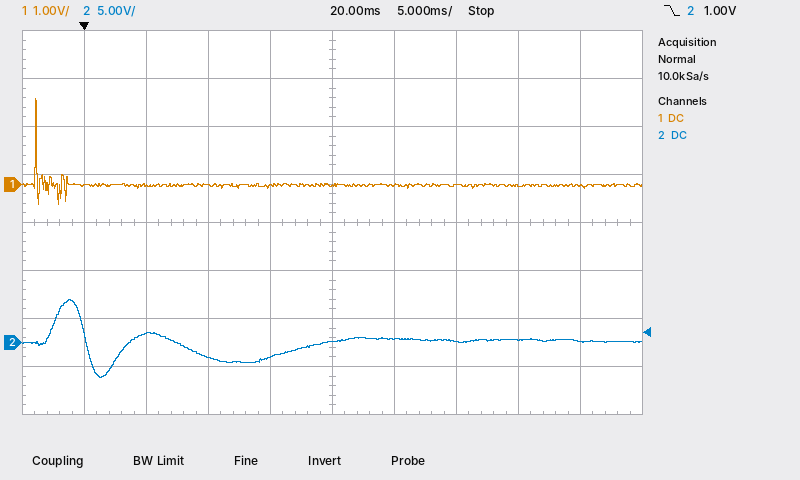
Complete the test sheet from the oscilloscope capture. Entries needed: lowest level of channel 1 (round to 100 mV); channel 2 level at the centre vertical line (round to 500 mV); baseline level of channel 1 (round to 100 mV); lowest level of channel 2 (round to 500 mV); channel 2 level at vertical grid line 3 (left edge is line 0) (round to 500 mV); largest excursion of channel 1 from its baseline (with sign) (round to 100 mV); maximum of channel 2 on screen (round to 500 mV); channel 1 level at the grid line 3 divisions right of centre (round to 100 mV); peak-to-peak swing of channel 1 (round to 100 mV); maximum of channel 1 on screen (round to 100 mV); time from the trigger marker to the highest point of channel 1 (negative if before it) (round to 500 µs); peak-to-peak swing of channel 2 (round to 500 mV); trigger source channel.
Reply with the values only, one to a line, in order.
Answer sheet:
-400 mV
0.0 V
0.0 V
-3.5 V
-1.5 V
+1.8 V
4.5 V
0.0 V
2.2 V
1.8 V
-4.0 ms
8.0 V
channel 2
